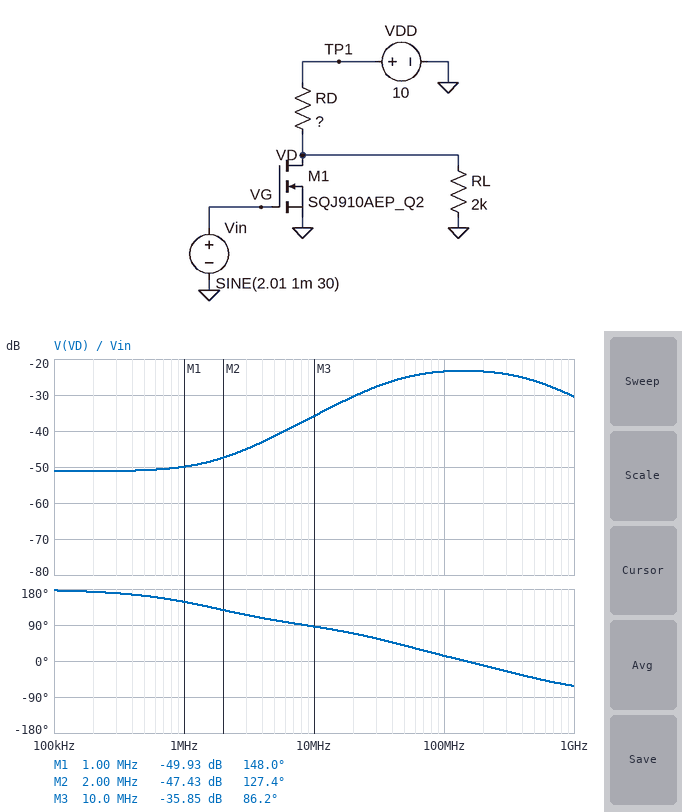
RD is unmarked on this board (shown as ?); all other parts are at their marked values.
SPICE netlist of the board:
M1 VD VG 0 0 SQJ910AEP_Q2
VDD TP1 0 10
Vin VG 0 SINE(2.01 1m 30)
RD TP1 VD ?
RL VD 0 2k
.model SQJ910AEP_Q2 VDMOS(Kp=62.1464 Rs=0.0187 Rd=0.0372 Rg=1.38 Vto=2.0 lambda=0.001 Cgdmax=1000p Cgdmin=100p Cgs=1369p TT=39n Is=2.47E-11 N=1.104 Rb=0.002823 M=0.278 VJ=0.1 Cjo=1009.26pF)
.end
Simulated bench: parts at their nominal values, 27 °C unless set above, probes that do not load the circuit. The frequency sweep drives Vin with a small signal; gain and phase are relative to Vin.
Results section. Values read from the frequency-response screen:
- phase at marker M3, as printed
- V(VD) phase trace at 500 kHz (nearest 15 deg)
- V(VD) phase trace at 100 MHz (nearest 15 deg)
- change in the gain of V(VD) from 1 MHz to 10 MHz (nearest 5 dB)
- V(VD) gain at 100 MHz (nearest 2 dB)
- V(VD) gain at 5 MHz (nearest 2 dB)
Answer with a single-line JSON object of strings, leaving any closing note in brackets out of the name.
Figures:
{"phase at marker M3, as printed": "86.2 deg", "V(VD) phase trace at 500 kHz": "165 deg", "V(VD) phase trace at 100 MHz": "15 deg", "change in the gain of V(VD) from 1 MHz to 10 MHz": "15 dB", "V(VD) gain at 100 MHz": "-24 dB", "V(VD) gain at 5 MHz": "-42 dB"}
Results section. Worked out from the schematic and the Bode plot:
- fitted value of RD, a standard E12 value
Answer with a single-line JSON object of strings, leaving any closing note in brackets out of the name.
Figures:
{"fitted value of RD, a standard E12 value": "5.6 kΩ"}
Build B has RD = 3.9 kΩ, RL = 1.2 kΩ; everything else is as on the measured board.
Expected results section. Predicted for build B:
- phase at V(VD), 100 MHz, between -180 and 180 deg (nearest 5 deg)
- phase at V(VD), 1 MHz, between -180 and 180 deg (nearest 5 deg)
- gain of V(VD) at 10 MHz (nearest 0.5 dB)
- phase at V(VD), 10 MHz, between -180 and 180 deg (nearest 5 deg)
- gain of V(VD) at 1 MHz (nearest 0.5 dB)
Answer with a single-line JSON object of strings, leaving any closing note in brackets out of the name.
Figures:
{"phase at V(VD), 100 MHz, between -180 and 180 deg": "15 deg", "phase at V(VD), 1 MHz, between -180 and 180 deg": "155 deg", "gain of V(VD) at 10 MHz": "-35.5 dB", "phase at V(VD), 10 MHz, between -180 and 180 deg": "90 deg", "gain of V(VD) at 1 MHz": "-47.5 dB"}
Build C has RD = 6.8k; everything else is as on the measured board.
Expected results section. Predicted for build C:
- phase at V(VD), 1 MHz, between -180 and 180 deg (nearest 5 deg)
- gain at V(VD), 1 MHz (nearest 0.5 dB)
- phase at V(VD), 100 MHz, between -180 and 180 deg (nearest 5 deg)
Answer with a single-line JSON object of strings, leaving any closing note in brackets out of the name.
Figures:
{"phase at V(VD), 1 MHz, between -180 and 180 deg": "145 deg", "gain at V(VD), 1 MHz": "-51.0 dB", "phase at V(VD), 100 MHz, between -180 and 180 deg": "15 deg"}
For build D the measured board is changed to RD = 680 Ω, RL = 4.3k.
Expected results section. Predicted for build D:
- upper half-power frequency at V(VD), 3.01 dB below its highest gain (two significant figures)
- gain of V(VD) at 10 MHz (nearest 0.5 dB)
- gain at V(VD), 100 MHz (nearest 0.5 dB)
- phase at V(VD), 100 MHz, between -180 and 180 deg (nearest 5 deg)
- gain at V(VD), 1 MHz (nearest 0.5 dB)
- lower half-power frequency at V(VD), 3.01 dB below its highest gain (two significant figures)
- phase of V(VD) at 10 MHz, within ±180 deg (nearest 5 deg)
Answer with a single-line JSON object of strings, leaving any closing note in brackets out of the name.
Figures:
{"upper half-power frequency at V(VD), 3.01 dB below its highest gain": "500 MHz", "gain of V(VD) at 10 MHz": "-31.0 dB", "gain at V(VD), 100 MHz": "-23.0 dB", "phase at V(VD), 100 MHz, between -180 and 180 deg": "20 deg", "gain at V(VD), 1 MHz": "-32.5 dB", "lower half-power frequency at V(VD), 3.01 dB below its highest gain": "34 MHz", "phase of V(VD) at 10 MHz, within ±180 deg": "130 deg"}
